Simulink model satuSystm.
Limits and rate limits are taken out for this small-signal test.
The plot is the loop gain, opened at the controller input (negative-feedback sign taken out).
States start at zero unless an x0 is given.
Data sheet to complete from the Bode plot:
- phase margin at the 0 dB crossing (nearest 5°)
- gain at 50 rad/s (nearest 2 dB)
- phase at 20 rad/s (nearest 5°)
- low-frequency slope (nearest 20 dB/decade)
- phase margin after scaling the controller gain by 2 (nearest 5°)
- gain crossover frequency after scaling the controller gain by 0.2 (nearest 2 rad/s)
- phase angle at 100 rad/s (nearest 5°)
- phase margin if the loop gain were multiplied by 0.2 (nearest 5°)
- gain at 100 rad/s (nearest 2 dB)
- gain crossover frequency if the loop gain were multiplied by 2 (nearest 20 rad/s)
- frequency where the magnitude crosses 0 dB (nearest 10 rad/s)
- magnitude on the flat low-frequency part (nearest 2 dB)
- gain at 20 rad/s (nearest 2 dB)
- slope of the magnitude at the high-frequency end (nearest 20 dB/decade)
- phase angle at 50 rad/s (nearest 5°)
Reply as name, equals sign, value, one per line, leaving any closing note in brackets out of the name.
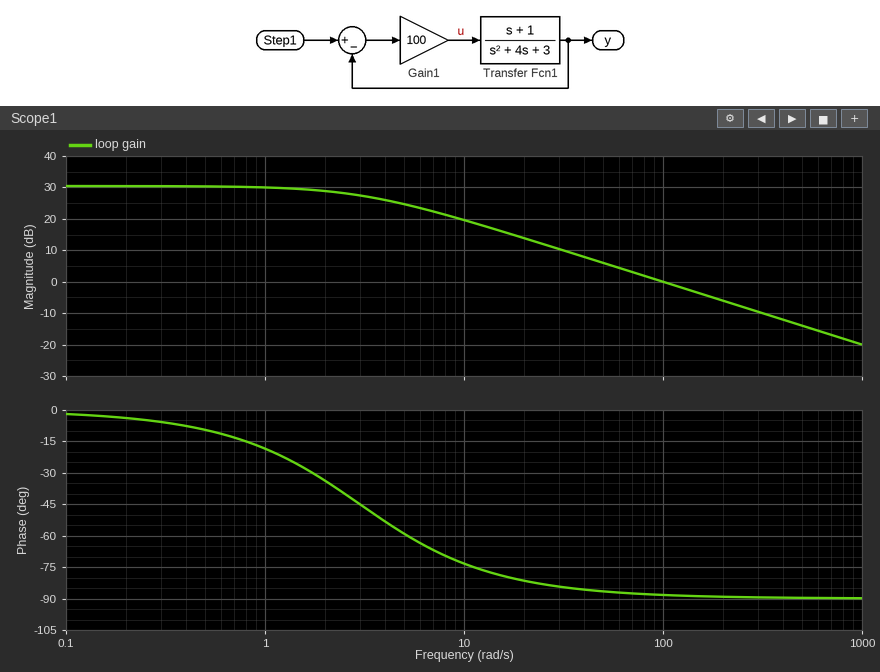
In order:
phase margin at the 0 dB crossing = 90°
gain at 50 rad/s = 6 dB
phase at 20 rad/s = -80°
low-frequency slope = 0 dB/decade
phase margin after scaling the controller gain by 2 = 90°
gain crossover frequency after scaling the controller gain by 0.2 = 20 rad/s
phase angle at 100 rad/s = -90°
phase margin if the loop gain were multiplied by 0.2 = 100°
gain at 100 rad/s = 0 dB
gain crossover frequency if the loop gain were multiplied by 2 = 200 rad/s
frequency where the magnitude crosses 0 dB = 100 rad/s
magnitude on the flat low-frequency part = 30 dB
gain at 20 rad/s = 14 dB
slope of the magnitude at the high-frequency end = -20 dB/decade
phase angle at 50 rad/s = -85°
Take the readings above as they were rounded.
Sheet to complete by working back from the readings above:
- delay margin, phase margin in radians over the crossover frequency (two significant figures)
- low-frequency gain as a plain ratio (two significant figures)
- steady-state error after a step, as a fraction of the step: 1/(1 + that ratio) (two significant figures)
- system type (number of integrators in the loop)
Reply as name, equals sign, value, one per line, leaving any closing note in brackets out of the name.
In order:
delay margin, phase margin in radians over the crossover frequency = 0.016 s
low-frequency gain as a plain ratio = 32
steady-state error after a step, as a fraction of the step: 1/(1 + that ratio) = 0.030
system type = 0
